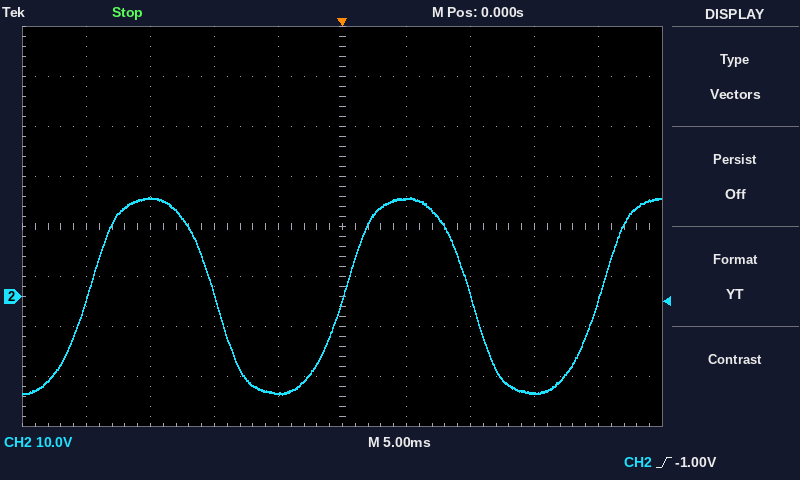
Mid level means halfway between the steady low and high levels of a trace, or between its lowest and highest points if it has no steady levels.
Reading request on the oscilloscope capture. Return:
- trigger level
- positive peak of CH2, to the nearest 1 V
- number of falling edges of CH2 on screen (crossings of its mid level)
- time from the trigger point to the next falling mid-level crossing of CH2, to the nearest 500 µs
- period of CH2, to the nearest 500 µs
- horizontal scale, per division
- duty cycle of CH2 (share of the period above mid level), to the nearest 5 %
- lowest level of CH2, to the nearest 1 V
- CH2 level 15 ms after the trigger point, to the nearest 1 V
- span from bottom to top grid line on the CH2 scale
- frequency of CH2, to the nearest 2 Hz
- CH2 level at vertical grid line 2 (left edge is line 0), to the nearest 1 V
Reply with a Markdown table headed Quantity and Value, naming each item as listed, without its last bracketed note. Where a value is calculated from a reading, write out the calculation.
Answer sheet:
| Quantity | Value |
|---|---|
| trigger level | -1.00 V |
| positive peak of CH2, to the nearest 1 V | 20 V |
| number of falling edges of CH2 on screen | 2 |
| time from the trigger point to the next falling mid-level crossing of CH2, to the nearest 500 µs | 10.0 ms |
| period of CH2, to the nearest 500 µs | 20.0 ms |
| horizontal scale, per division | 5 ms |
| duty cycle of CH2 (share of the period above mid level), to the nearest 5 % | 50 % |
| lowest level of CH2, to the nearest 1 V | -20 V |
| CH2 level 15 ms after the trigger point, to the nearest 1 V | -19 V |
| span from bottom to top grid line on the CH2 scale | 80 V |
| frequency of CH2, to the nearest 2 Hz | 1 / 20.0 ms ≈ 50 Hz |
| CH2 level at vertical grid line 2 (left edge is line 0), to the nearest 1 V | 20 V |
